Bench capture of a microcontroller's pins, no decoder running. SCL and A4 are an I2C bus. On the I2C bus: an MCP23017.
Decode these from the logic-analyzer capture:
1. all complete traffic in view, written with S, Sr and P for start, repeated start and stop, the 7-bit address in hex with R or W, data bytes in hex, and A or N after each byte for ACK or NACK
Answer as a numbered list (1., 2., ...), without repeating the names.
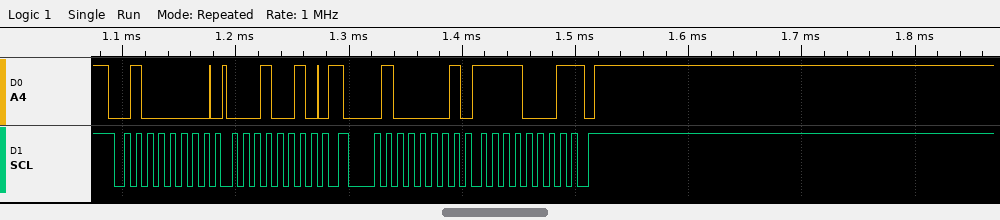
1. S 20W A 12 A Sr 20R A F1 N P
